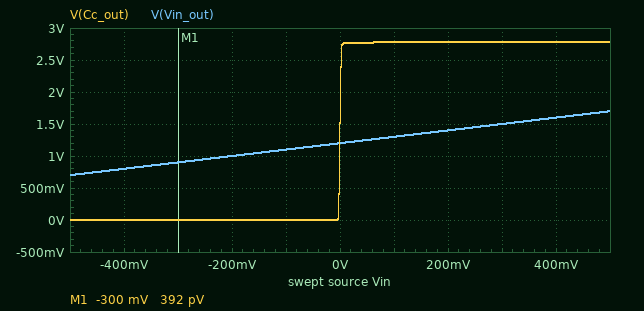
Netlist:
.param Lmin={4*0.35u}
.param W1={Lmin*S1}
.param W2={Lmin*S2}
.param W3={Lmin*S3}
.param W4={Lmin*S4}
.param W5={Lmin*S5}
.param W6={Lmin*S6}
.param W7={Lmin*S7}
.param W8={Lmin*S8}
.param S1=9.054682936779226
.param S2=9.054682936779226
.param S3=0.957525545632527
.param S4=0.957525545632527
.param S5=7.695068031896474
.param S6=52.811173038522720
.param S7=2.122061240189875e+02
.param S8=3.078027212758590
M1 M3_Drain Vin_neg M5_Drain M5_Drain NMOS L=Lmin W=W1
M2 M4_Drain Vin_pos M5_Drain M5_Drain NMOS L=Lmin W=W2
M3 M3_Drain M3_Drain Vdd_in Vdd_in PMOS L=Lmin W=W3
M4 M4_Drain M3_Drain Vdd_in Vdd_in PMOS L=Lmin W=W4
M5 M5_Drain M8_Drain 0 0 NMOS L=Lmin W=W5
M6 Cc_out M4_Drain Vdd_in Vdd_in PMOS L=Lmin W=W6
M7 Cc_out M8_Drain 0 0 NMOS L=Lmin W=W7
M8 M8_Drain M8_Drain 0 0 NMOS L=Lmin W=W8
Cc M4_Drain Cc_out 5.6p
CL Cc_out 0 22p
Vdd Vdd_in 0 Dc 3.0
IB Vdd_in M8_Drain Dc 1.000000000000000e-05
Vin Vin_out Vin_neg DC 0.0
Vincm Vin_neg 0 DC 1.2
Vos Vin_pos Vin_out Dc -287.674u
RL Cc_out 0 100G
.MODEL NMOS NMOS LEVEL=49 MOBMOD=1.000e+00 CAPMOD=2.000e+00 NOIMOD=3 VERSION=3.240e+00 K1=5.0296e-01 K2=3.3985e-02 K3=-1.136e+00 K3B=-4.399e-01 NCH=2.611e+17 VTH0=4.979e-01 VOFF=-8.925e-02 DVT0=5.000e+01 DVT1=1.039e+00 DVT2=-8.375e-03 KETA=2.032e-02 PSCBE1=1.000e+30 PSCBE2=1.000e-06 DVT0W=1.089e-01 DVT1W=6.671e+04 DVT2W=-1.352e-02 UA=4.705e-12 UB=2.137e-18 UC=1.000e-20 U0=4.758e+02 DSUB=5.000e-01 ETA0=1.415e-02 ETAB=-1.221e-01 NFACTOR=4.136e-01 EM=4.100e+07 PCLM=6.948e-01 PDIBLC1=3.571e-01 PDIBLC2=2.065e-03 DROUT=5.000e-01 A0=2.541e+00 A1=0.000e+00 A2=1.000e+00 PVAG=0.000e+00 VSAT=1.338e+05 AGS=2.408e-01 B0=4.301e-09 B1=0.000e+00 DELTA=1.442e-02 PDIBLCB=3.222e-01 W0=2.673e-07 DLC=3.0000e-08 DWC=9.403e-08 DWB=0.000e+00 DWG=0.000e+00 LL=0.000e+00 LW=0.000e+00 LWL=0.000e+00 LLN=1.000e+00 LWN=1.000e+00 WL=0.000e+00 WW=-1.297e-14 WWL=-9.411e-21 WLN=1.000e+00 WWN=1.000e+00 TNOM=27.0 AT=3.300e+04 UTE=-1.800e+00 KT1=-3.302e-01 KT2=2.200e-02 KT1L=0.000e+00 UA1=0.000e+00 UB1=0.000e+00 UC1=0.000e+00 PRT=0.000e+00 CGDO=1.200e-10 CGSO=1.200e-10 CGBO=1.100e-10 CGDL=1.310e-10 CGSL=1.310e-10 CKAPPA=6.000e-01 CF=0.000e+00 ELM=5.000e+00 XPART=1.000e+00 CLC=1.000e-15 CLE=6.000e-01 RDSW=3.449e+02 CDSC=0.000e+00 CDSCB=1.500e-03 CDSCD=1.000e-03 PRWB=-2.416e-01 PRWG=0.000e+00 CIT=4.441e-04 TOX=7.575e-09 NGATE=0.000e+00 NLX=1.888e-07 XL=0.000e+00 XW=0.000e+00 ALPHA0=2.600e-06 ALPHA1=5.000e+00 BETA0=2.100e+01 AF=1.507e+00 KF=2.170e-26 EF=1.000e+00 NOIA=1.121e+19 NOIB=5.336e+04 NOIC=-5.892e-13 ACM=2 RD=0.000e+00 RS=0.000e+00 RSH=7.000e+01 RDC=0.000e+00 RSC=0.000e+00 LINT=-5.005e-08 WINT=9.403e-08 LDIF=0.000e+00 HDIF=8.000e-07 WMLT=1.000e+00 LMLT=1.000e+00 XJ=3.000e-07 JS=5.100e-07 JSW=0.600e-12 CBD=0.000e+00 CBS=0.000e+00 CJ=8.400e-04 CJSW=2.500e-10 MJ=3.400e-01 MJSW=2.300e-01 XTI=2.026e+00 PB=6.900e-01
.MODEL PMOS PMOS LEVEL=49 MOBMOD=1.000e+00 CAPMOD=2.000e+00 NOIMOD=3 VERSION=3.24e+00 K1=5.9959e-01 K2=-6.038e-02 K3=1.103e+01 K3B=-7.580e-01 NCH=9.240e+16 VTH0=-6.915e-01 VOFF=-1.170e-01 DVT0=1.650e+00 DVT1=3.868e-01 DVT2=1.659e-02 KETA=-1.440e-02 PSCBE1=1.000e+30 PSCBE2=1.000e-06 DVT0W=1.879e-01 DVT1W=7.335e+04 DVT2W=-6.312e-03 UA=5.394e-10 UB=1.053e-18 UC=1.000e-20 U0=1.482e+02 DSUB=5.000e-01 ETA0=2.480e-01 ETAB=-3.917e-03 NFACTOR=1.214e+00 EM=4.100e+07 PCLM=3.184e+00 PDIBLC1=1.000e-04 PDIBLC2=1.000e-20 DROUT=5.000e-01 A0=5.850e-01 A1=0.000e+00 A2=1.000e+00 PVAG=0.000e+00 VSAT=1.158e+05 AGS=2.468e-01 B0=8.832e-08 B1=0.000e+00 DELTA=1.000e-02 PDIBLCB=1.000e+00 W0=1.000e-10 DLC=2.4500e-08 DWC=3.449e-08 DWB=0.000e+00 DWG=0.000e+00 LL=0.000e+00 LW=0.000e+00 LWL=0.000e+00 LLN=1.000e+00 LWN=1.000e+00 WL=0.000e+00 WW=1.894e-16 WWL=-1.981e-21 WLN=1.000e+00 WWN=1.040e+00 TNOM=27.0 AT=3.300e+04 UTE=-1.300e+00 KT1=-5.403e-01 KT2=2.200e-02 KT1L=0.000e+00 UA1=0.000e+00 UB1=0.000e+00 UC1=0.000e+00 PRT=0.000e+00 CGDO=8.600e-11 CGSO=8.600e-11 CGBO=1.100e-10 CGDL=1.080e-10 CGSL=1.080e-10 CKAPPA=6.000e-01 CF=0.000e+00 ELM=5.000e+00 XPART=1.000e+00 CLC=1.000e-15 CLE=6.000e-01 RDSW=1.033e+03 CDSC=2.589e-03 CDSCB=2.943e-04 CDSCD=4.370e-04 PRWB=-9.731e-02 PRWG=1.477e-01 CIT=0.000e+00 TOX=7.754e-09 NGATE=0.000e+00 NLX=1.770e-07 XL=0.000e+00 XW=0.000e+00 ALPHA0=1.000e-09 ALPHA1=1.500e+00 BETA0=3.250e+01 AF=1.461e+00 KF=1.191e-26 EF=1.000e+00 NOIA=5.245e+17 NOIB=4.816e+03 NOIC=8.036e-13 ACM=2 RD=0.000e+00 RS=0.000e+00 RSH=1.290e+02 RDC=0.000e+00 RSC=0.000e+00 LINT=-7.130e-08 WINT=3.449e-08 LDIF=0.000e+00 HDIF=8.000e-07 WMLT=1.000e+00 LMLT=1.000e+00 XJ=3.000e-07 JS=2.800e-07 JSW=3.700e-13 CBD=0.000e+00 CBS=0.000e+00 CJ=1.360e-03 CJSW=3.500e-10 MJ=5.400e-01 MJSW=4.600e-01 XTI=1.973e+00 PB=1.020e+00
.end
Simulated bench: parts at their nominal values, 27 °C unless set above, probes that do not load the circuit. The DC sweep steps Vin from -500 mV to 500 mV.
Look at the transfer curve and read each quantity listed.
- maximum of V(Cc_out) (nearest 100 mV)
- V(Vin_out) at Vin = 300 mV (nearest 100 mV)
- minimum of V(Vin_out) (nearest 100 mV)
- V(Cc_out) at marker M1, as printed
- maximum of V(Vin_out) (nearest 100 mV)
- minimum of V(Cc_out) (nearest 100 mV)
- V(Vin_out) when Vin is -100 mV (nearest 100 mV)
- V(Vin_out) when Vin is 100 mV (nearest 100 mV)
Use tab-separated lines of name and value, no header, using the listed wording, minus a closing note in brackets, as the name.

maximum of V(Cc_out)	2.8 V
V(Vin_out) at Vin = 300 mV	1.5 V
minimum of V(Vin_out)	700 mV
V(Cc_out) at marker M1, as printed	392 pV
maximum of V(Vin_out)	1.7 V
minimum of V(Cc_out)	0 V
V(Vin_out) when Vin is -100 mV	1.1 V
V(Vin_out) when Vin is 100 mV	1.3 V
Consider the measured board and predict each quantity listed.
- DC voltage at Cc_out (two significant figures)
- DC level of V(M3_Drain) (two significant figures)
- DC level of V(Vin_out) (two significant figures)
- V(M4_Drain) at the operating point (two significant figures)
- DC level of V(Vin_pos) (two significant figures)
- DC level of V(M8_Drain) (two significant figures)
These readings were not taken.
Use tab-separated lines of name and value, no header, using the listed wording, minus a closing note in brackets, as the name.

DC voltage at Cc_out	1.5 V
DC level of V(M3_Drain)	1.4 V
DC level of V(Vin_out)	1.2 V
V(M4_Drain) at the operating point	1.5 V
DC level of V(Vin_pos)	1.2 V
DC level of V(M8_Drain)	740 mV
